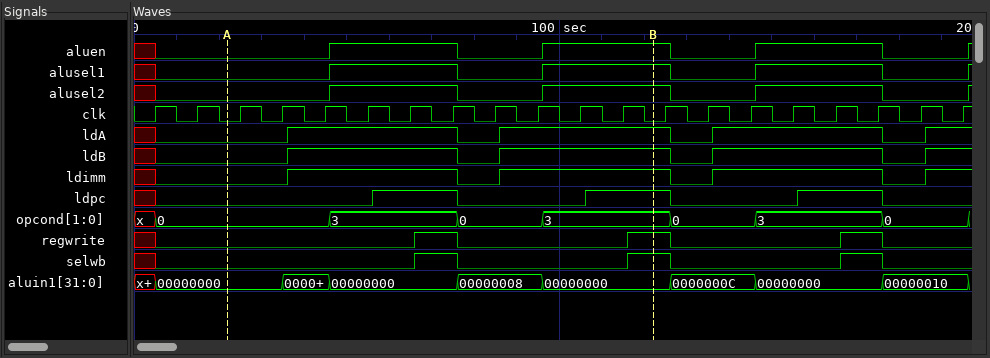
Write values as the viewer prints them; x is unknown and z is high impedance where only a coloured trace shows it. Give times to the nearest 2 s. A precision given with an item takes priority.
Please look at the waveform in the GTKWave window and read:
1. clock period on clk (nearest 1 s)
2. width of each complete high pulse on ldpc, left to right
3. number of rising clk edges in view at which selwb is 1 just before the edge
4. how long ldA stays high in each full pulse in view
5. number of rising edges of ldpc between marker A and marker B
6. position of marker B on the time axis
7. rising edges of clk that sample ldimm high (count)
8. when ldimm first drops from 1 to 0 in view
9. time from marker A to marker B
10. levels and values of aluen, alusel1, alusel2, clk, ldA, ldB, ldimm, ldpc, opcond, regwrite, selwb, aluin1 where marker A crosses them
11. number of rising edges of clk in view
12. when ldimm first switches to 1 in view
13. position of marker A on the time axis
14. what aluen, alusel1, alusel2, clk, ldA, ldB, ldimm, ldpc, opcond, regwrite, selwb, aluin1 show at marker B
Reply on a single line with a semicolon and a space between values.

10 s; 20 s, 20 s, 20 s; 3; 40 s, 40 s, 40 s; 2; 122 s; 13; 76 s; 100 s; aluen=0, alusel1=0, alusel2=0, clk=0, ldA=0, ldB=0, ldimm=0, ldpc=0, opcond=0, regwrite=0, selwb=0, aluin1=00000000; 20; 36 s; 22 s; aluen=1, alusel1=1, alusel2=1, clk=0, ldA=1, ldB=1, ldimm=1, ldpc=1, opcond=3, regwrite=1, selwb=1, aluin1=00000000
